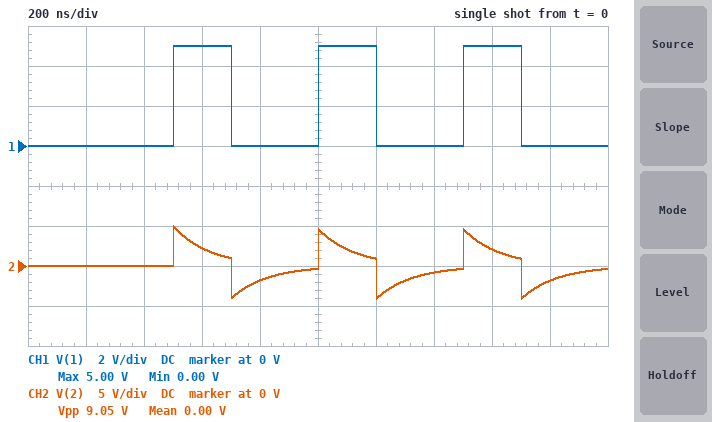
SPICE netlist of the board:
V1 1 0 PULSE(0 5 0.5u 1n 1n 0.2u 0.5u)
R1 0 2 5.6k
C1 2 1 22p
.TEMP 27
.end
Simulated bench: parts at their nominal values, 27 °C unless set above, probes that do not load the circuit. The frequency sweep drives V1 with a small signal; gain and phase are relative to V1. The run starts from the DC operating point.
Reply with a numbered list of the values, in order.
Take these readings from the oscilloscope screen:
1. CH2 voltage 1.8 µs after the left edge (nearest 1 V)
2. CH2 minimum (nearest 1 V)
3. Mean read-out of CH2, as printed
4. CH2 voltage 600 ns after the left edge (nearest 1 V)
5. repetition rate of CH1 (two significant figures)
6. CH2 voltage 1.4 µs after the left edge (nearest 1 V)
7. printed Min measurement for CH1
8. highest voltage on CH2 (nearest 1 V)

1. -2 V
2. -4 V
3. 0.00 V
4. 2 V
5. 2.0 MHz
6. -1 V
7. 0.00 V
8. 5 V
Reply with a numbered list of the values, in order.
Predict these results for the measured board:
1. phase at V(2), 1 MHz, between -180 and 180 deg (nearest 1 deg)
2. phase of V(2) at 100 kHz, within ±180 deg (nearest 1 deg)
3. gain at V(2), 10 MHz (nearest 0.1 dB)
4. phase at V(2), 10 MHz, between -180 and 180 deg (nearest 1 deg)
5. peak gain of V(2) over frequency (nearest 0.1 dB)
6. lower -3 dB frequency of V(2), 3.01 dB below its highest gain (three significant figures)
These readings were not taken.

1. 52 deg
2. 86 deg
3. -0.1 dB
4. 7 deg
5. 0 dB
6. 1.29 MHz
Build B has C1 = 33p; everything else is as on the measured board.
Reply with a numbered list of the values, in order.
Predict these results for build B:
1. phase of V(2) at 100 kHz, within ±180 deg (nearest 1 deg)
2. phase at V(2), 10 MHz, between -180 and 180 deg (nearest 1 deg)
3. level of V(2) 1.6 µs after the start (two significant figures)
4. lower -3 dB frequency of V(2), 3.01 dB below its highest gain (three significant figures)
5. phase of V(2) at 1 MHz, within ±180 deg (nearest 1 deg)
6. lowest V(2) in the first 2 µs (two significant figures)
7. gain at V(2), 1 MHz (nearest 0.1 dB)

1. 83 deg
2. 5 deg
3. 2.5 V
4. 861 kHz
5. 41 deg
6. -3.5 V
7. -2.4 dB
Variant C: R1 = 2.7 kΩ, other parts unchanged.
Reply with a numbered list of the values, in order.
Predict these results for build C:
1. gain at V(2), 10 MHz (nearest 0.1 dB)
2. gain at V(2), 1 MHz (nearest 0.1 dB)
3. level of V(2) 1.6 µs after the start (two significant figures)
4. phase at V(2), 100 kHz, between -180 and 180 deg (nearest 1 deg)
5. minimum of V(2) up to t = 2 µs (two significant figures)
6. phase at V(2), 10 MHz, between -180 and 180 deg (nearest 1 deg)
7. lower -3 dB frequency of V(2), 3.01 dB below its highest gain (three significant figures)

1. -0.3 dB
2. -9.1 dB
3. 930 mV
4. 88 deg
5. -4.8 V
6. 15 deg
7. 2.68 MHz
